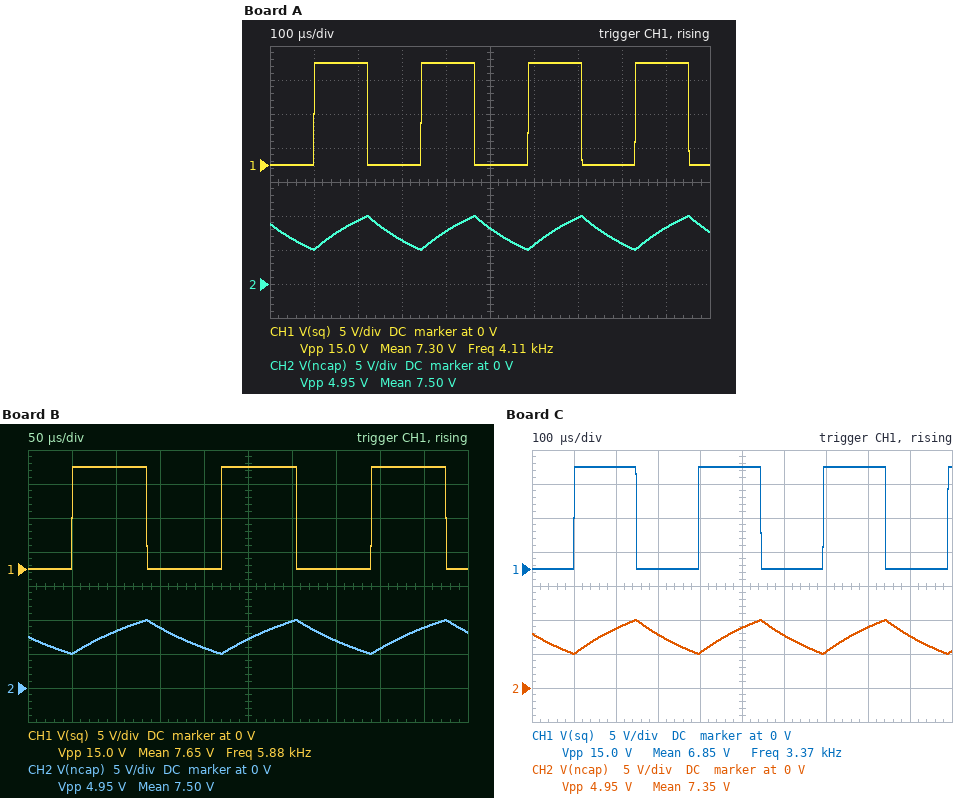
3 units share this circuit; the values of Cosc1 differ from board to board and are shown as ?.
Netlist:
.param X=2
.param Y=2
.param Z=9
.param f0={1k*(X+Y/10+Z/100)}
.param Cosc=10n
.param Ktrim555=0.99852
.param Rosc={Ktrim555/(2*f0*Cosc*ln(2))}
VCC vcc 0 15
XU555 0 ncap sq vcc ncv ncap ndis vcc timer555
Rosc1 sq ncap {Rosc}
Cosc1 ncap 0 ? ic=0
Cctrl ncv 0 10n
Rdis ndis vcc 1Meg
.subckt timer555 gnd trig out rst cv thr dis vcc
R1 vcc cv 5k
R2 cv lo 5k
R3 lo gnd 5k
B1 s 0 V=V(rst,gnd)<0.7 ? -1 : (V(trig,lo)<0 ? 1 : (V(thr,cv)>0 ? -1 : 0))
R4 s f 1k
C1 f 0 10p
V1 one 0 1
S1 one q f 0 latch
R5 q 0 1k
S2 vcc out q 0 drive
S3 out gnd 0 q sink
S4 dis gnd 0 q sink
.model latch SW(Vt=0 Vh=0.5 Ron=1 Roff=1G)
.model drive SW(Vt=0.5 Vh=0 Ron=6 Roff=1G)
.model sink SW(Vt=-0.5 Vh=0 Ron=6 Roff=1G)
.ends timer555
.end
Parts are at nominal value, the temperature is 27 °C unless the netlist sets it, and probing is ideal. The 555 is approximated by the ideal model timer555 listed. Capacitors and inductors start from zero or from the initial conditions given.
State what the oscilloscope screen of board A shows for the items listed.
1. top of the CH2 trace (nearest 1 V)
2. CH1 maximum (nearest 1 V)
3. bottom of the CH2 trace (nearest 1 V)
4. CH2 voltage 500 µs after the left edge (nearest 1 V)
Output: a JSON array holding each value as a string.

["10 V", "15 V", "5 V", "8 V"]
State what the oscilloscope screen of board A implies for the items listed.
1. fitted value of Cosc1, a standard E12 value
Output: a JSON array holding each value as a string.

["5.6 nF"]
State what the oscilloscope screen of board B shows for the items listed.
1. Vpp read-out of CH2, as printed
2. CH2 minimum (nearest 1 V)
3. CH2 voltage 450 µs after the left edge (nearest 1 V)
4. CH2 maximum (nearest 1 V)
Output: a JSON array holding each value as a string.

["4.95 V", "5 V", "9 V", "10 V"]
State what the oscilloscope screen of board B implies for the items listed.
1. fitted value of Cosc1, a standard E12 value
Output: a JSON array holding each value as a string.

["3.9 nF"]
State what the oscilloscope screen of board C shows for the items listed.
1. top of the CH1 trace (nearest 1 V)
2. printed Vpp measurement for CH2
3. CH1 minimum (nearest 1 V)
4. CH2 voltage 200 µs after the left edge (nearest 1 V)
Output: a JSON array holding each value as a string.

["15 V", "4.95 V", "0 V", "9 V"]
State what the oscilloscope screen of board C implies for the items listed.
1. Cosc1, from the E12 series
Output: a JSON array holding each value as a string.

["6.8 nF"]
